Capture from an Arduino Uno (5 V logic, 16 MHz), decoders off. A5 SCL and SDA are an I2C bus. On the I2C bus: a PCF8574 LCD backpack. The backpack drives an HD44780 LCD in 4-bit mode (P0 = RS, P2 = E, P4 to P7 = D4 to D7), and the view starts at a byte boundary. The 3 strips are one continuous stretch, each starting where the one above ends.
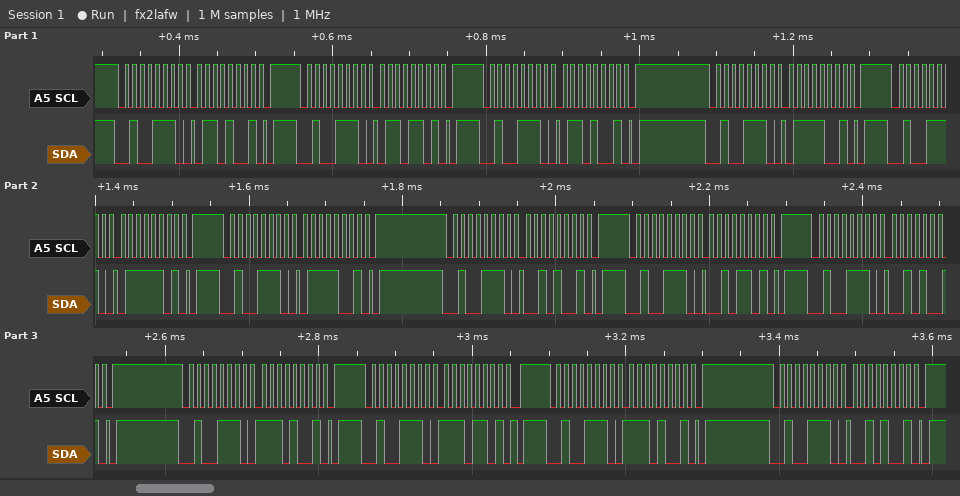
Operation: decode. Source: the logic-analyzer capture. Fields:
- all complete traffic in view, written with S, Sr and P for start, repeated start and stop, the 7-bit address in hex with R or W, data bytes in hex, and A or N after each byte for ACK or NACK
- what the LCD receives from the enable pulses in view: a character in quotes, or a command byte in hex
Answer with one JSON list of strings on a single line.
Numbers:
["S 27W A 69 A P S 27W A 6D A P S 27W A 69 A P S 27W A 79 A P S 27W A 7D A P S 27W A 79 A P S 27W A 29 A P S 27W A 2D A P S 27W A 29 A P S 27W A E9 A P S 27W A ED A P S 27W A E9 A P S 27W A 29 A P", "'g' '.'"]
